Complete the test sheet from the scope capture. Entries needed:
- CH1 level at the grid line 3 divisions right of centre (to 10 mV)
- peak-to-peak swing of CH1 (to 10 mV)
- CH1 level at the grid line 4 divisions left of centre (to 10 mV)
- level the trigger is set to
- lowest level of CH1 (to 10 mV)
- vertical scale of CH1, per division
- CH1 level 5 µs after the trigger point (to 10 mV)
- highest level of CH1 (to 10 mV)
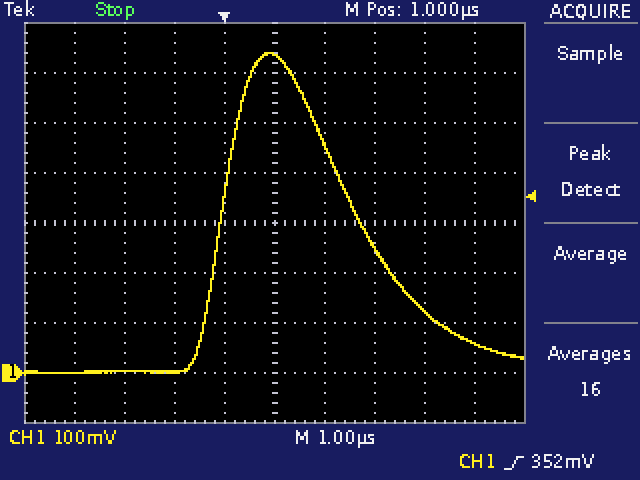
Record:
120 mV
640 mV
0 mV
352 mV
0 mV
100 mV
60 mV
640 mV
